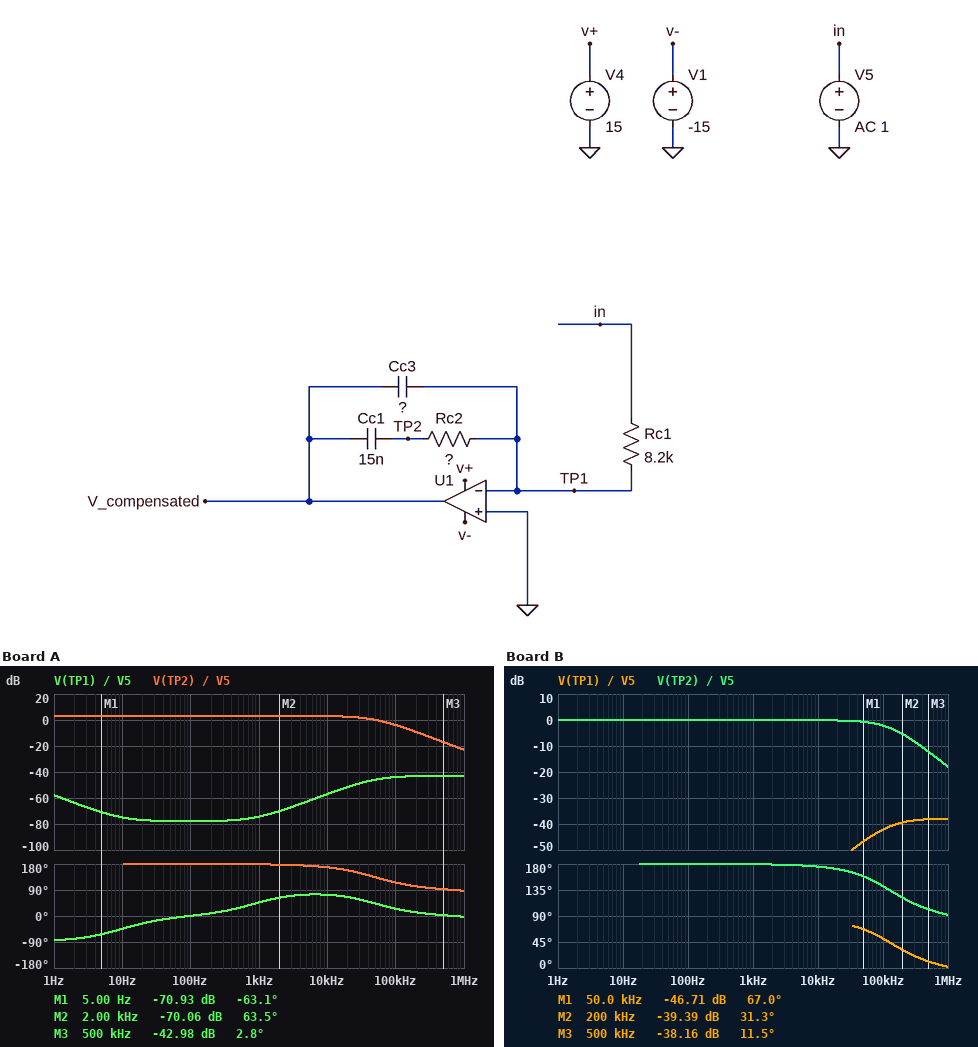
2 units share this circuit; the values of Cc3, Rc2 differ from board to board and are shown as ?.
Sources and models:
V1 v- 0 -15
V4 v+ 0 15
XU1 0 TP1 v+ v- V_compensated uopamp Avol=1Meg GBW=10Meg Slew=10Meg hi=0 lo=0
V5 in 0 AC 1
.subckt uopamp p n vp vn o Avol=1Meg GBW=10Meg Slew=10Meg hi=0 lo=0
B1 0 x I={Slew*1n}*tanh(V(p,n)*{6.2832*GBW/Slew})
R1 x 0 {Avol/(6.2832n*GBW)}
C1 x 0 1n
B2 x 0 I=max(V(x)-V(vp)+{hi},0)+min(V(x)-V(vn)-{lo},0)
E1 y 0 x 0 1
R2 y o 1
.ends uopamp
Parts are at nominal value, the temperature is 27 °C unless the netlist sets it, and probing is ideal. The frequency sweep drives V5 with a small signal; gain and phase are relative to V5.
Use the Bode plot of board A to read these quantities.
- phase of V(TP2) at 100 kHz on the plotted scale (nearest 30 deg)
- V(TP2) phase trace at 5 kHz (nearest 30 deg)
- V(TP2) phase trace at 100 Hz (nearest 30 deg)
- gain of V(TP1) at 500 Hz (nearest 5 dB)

120 deg
180 deg
180 deg
-75 dB
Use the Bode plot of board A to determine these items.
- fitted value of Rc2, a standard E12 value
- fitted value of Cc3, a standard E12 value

12 kΩ
270 pF
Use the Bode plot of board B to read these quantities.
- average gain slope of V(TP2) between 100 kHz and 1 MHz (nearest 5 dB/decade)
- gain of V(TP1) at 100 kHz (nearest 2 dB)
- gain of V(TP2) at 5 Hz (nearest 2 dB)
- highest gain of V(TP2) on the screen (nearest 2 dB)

-15 dB/decade
-42 dB
0 dB
0 dB
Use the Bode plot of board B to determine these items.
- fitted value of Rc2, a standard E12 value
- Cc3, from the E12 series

8.2 kΩ
150 pF
